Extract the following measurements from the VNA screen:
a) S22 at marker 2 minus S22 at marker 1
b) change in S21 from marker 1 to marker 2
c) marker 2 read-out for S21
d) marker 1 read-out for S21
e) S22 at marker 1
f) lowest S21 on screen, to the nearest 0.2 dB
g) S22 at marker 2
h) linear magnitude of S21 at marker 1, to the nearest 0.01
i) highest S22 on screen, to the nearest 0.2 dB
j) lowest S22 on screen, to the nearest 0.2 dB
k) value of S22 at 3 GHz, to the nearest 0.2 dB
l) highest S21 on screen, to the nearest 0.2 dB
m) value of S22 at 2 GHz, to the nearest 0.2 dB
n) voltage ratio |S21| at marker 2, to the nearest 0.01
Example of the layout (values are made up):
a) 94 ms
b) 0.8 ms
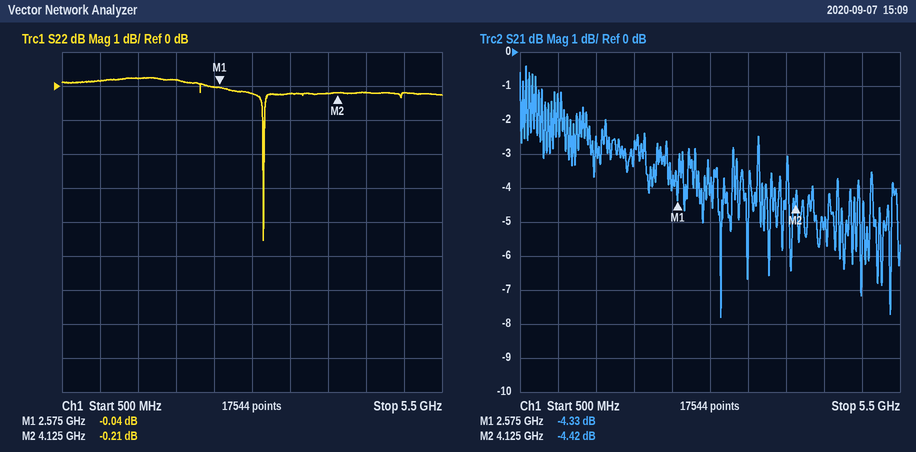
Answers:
a) -0.17 dB
b) -0.09 dB
c) -4.42 dB
d) -4.33 dB
e) -0.04 dB
f) -7.8 dB
g) -0.21 dB
h) 0.61
i) 0.2 dB
j) -4.6 dB
k) -0.2 dB
l) -0.4 dB
m) 0.2 dB
n) 0.60
